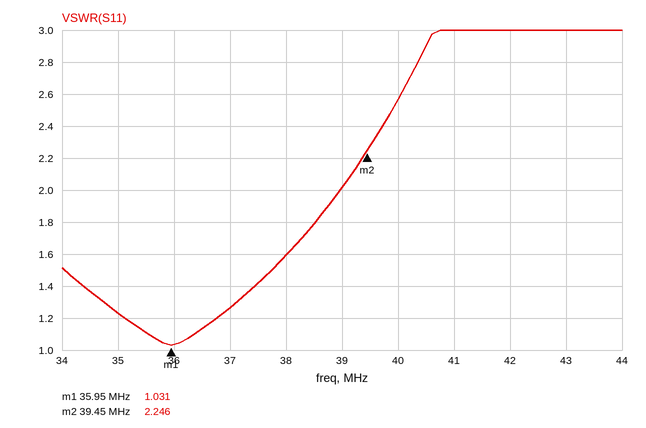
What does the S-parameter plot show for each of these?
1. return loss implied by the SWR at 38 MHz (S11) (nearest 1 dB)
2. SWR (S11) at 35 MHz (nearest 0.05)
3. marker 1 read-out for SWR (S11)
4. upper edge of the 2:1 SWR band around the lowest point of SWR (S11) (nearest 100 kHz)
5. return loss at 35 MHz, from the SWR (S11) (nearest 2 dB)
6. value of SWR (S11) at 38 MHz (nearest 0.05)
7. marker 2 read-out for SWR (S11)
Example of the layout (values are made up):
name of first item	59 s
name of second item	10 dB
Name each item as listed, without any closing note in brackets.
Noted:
return loss implied by the SWR at 38 MHz (S11)	13 dB
SWR (S11) at 35 MHz	1.25
marker 1 read-out for SWR	1.031
upper edge of the 2:1 SWR band around the lowest point of SWR (S11)	39.0 MHz
return loss at 35 MHz, from the SWR (S11)	20 dB
value of SWR (S11) at 38 MHz	1.60
marker 2 read-out for SWR	2.246
